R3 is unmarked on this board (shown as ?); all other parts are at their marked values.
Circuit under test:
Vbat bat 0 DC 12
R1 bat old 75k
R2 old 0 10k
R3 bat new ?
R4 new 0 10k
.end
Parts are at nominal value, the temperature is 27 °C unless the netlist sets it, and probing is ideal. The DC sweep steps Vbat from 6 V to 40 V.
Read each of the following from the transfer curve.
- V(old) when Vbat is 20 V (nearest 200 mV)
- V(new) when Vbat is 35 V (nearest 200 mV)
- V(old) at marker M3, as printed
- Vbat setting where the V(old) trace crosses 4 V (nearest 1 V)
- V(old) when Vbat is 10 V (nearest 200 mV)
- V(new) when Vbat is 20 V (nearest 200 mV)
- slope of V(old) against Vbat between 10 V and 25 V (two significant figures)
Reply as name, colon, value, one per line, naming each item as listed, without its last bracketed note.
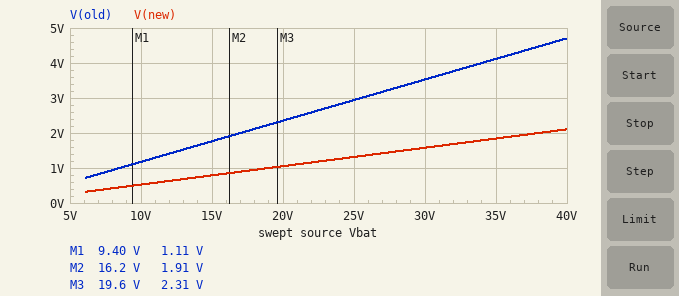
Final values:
V(old) when Vbat is 20 V: 2.4 V
V(new) when Vbat is 35 V: 1.8 V
V(old) at marker M3, as printed: 2.31 V
Vbat setting where the V(old) trace crosses 4 V: 34 V
V(old) when Vbat is 10 V: 1.2 V
V(new) when Vbat is 20 V: 1.0 V
slope of V(old) against Vbat between 10 V and 25 V: 0.12 V/V
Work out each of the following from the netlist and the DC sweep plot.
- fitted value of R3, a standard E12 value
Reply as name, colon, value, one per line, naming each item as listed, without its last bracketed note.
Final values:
fitted value of R3, a standard E12 value: 180 kΩ
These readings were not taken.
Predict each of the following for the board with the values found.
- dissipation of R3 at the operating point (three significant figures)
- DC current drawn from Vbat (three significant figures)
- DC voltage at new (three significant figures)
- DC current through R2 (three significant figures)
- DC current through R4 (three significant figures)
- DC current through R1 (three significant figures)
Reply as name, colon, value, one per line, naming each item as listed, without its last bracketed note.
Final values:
dissipation of R3 at the operating point: 718 µW
DC current drawn from Vbat: 204 µA
DC voltage at new: 632 mV
DC current through R2: 141 µA
DC current through R4: 63.2 µA
DC current through R1: 141 µA
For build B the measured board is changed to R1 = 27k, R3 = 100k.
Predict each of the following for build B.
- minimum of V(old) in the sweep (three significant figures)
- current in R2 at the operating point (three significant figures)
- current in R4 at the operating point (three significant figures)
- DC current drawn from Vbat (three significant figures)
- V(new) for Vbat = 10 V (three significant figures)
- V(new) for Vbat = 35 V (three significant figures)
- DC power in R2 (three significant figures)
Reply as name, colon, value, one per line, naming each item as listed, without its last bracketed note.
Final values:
minimum of V(old) in the sweep: 1.62 V
current in R2 at the operating point: 324 µA
current in R4 at the operating point: 109 µA
DC current drawn from Vbat: 433 µA
V(new) for Vbat = 10 V: 909 mV
V(new) for Vbat = 35 V: 3.18 V
DC power in R2: 1.05 mW
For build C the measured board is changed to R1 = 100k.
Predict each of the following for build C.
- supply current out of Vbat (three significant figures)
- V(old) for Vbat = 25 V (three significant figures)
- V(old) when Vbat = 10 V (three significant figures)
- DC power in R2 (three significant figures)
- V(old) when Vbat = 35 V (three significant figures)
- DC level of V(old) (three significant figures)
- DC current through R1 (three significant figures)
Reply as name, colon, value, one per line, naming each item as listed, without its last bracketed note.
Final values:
supply current out of Vbat: 172 µA
V(old) for Vbat = 25 V: 2.27 V
V(old) when Vbat = 10 V: 909 mV
DC power in R2: 119 µW
V(old) when Vbat = 35 V: 3.18 V
DC level of V(old): 1.09 V
DC current through R1: 109 µA
